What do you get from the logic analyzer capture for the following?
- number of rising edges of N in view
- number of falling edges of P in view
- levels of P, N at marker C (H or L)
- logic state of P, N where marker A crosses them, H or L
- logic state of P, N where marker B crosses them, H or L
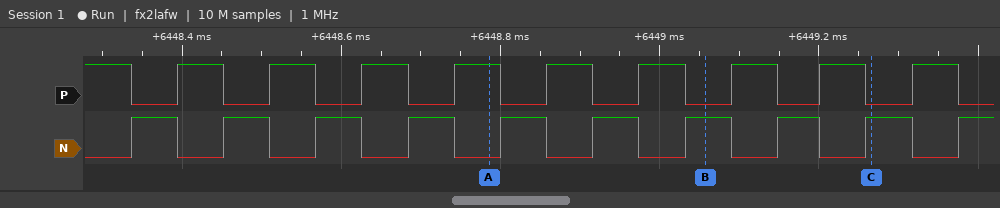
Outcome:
10
10
P=L, N=H
P=H, N=L
P=L, N=H
